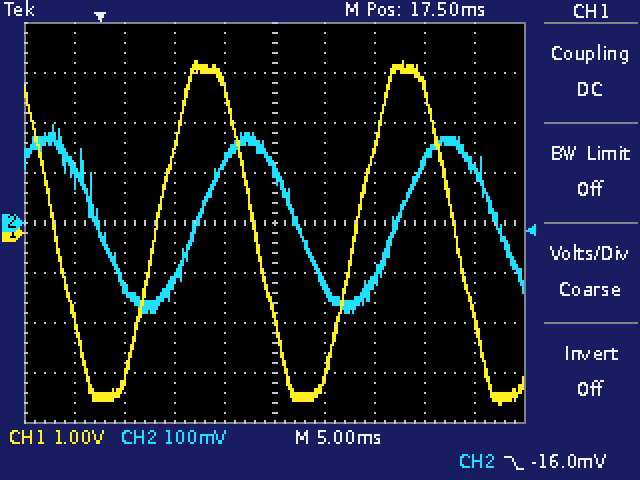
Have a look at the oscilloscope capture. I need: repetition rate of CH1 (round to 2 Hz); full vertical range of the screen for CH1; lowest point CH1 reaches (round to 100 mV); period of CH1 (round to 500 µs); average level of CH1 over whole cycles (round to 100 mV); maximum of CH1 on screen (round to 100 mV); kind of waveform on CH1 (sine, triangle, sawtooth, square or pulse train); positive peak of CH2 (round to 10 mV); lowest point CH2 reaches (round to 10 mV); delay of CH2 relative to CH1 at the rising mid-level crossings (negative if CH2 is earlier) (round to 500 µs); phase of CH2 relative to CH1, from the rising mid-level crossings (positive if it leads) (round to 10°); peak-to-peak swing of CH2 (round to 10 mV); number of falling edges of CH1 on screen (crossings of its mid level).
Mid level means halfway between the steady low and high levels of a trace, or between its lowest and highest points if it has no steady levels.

50 Hz
8 V
-3.4 V
20.0 ms
0.0 V
3.4 V
sine
200 mV
-180 mV
+4.5 ms
-80°
380 mV
3
